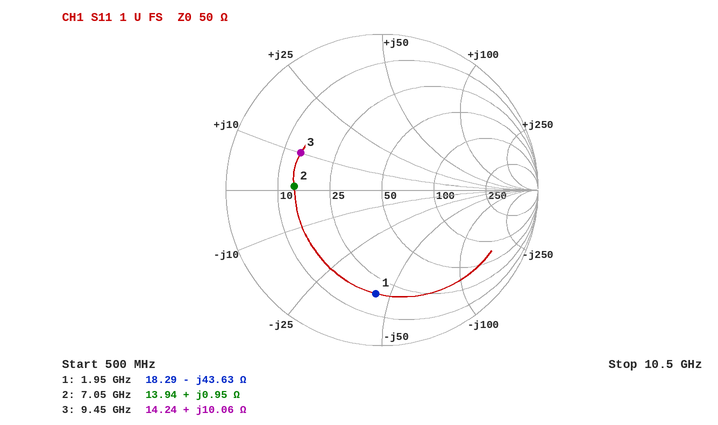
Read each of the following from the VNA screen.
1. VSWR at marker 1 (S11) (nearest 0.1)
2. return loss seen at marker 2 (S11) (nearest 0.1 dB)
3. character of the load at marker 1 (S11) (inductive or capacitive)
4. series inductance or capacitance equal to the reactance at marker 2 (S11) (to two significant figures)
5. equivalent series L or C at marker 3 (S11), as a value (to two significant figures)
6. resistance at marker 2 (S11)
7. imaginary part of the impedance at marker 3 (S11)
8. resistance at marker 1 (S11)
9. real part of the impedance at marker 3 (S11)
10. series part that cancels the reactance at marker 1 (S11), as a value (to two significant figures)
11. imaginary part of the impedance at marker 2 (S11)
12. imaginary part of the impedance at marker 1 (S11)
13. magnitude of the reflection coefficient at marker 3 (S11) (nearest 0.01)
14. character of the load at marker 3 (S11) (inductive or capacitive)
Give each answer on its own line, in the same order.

5.0
5.0 dB
capacitive
21 pH
170 pH
13.94 Ω
+10.06 Ω
18.29 Ω
14.24 Ω
3.6 nH
+0.95 Ω
-43.63 Ω
0.57
inductive
